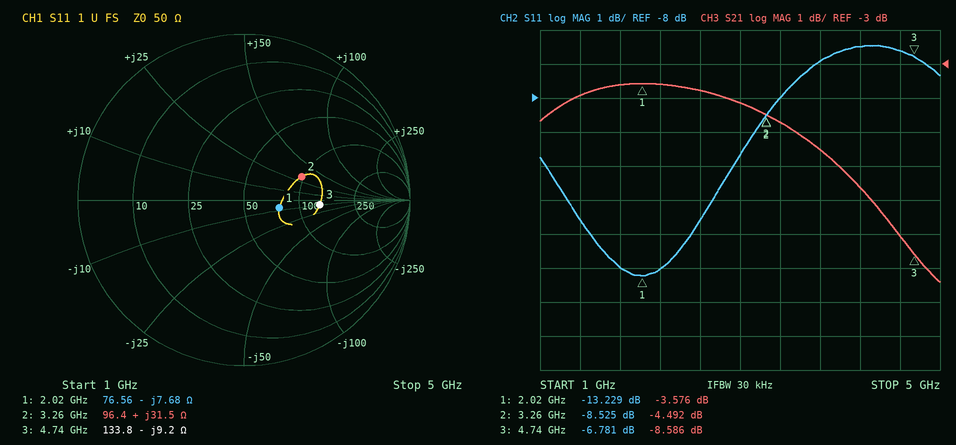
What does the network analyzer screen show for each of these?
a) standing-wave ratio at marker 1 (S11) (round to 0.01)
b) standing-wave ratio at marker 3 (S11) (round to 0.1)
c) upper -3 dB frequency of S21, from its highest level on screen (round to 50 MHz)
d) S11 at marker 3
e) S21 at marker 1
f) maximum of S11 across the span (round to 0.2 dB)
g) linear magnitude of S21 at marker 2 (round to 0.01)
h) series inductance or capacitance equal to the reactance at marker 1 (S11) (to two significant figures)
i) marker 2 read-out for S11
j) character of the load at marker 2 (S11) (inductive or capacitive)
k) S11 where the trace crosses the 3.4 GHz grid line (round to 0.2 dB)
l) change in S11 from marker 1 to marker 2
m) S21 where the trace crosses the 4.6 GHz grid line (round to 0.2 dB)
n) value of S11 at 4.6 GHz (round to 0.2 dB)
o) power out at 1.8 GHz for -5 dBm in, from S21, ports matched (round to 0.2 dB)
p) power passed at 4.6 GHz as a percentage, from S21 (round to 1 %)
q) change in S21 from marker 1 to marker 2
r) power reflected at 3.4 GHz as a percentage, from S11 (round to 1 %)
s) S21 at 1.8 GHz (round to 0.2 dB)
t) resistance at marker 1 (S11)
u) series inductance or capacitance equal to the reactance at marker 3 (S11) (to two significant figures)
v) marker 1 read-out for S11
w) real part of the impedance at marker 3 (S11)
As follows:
1.56
2.7
4.20 GHz
-6.781 dB
-3.576 dB
-6.4 dB
0.60
10 pF
-8.525 dB
inductive
-8.0 dB
4.704 dB
-8.0 dB
-6.6 dB
-8.6 dBm
16 %
-0.916 dB
16 %
-3.6 dB
76.56 Ω
3.6 pF
-13.229 dB
133.8 Ω
